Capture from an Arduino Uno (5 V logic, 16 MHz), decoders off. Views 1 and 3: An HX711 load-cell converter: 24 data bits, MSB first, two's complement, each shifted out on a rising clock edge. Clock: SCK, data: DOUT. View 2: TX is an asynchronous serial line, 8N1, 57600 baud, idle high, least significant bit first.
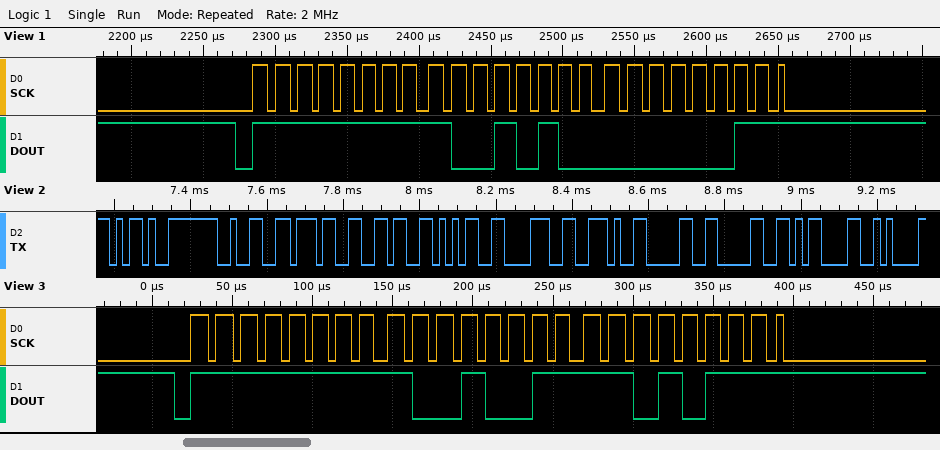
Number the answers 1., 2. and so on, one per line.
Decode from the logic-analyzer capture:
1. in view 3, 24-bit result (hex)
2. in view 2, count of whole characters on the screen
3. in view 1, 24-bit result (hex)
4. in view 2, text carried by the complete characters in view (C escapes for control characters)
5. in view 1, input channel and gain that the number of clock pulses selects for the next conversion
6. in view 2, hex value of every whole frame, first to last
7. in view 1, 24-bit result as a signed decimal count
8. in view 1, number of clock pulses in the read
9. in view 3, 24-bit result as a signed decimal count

1. 0xFF93D7
2. 11
3. 0xFF9403
4. "-27658.00\r\n"
5. channel A, gain 128
6. 2D 32 37 36 35 38 2E 30 30 0D 0A
7. -27645
8. 25
9. -27689
